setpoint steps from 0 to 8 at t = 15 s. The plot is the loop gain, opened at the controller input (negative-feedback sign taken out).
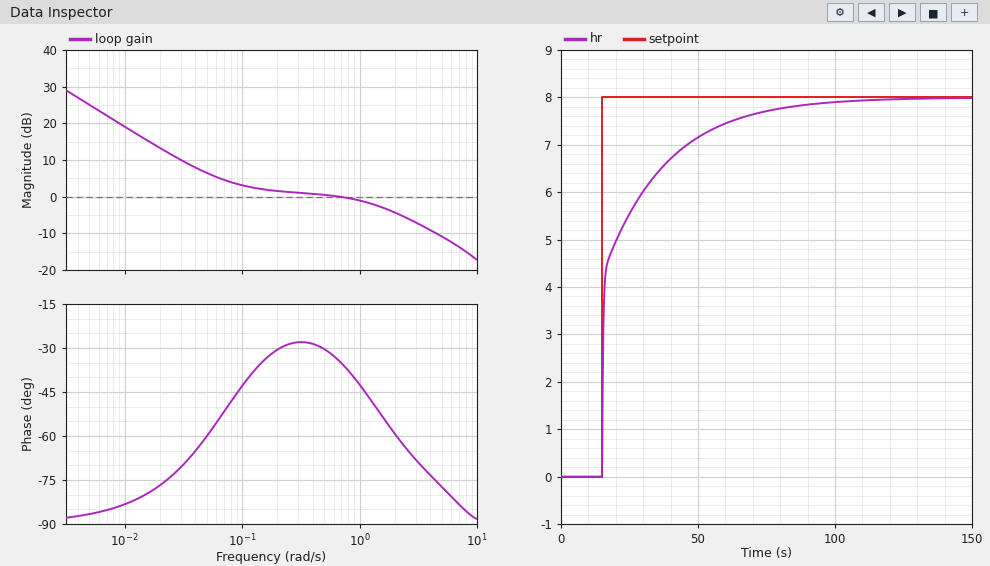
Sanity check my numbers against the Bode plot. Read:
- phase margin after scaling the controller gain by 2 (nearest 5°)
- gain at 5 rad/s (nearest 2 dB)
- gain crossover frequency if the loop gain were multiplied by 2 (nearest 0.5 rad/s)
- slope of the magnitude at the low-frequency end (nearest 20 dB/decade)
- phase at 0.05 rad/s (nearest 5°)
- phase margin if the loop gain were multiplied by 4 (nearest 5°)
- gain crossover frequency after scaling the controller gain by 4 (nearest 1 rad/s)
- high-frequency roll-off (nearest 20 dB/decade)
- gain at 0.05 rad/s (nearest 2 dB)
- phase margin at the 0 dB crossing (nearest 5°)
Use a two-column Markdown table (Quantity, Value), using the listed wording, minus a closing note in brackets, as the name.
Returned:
| Quantity | Value |
|---|---|
| phase margin after scaling the controller gain by 2 | 115° |
| gain at 5 rad/s | -10 dB |
| gain crossover frequency if the loop gain were multiplied by 2 | 2.5 rad/s |
| slope of the magnitude at the low-frequency end | -20 dB/decade |
| phase at 0.05 rad/s | -60° |
| phase margin if the loop gain were multiplied by 4 | 100° |
| gain crossover frequency after scaling the controller gain by 4 | 6 rad/s |
| high-frequency roll-off | -20 dB/decade |
| gain at 0.05 rad/s | 6 dB |
| phase margin at the 0 dB crossing | 145° |
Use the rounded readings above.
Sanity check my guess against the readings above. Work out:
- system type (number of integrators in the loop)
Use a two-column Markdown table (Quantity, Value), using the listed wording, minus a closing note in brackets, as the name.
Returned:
| Quantity | Value |
|---|---|
| system type | 1 |
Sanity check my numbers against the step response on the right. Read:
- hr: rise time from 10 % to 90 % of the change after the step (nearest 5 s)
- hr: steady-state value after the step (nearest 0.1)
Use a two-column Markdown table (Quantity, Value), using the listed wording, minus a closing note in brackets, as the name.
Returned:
| Quantity | Value |
|---|---|
| hr: rise time from 10 % to 90 % of the change after the step | 35 s |
| hr: steady-state value after the step | 8.0 |
